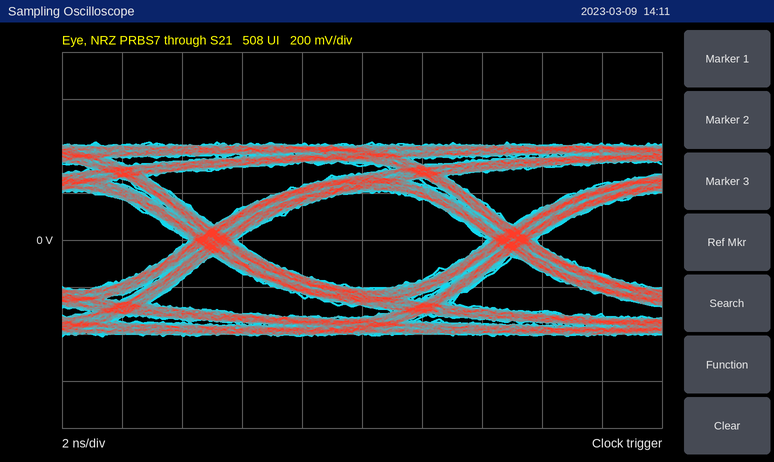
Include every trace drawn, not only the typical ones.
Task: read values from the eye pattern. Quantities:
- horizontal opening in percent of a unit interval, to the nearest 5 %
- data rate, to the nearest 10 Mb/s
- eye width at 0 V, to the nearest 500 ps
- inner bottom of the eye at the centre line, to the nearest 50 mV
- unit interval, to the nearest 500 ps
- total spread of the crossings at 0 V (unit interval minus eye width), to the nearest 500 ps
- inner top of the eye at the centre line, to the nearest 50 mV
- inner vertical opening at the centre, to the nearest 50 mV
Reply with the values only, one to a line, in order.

85 %
100 Mb/s
8.5 ns
-200 mV
10.0 ns
1.5 ns
200 mV
400 mV
